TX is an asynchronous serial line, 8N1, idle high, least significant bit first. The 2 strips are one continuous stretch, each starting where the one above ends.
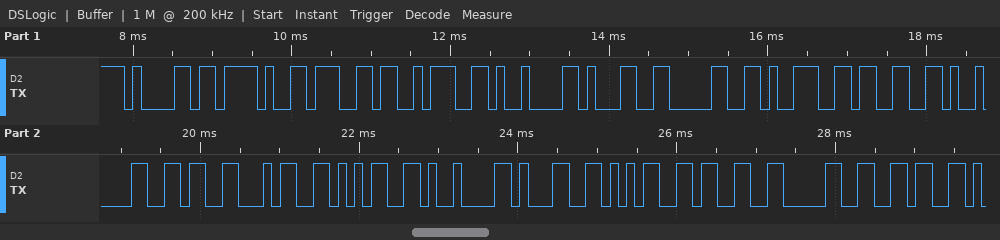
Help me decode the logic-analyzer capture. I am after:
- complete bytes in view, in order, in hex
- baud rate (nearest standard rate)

0x61 0x2F 0x67 0x3A 0x09 0x31 0x30 0x39 0x33 0x09 0x36 0x34 0x35 0x09 0x31 0x35 0x33 0x30 0x36
9600 baud
